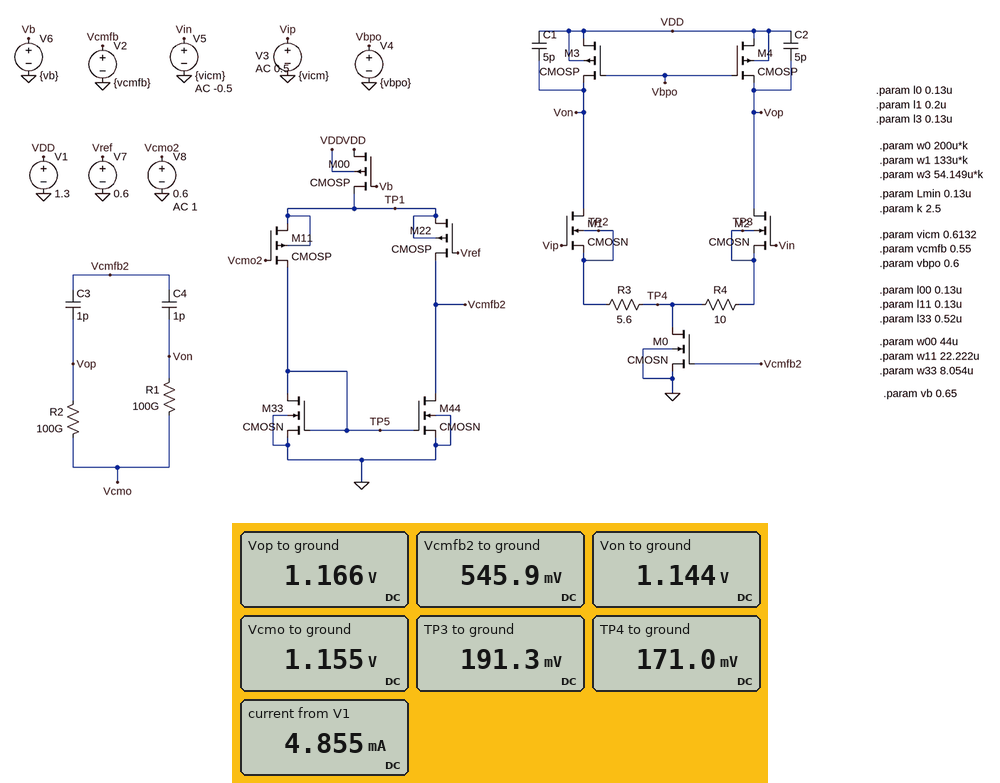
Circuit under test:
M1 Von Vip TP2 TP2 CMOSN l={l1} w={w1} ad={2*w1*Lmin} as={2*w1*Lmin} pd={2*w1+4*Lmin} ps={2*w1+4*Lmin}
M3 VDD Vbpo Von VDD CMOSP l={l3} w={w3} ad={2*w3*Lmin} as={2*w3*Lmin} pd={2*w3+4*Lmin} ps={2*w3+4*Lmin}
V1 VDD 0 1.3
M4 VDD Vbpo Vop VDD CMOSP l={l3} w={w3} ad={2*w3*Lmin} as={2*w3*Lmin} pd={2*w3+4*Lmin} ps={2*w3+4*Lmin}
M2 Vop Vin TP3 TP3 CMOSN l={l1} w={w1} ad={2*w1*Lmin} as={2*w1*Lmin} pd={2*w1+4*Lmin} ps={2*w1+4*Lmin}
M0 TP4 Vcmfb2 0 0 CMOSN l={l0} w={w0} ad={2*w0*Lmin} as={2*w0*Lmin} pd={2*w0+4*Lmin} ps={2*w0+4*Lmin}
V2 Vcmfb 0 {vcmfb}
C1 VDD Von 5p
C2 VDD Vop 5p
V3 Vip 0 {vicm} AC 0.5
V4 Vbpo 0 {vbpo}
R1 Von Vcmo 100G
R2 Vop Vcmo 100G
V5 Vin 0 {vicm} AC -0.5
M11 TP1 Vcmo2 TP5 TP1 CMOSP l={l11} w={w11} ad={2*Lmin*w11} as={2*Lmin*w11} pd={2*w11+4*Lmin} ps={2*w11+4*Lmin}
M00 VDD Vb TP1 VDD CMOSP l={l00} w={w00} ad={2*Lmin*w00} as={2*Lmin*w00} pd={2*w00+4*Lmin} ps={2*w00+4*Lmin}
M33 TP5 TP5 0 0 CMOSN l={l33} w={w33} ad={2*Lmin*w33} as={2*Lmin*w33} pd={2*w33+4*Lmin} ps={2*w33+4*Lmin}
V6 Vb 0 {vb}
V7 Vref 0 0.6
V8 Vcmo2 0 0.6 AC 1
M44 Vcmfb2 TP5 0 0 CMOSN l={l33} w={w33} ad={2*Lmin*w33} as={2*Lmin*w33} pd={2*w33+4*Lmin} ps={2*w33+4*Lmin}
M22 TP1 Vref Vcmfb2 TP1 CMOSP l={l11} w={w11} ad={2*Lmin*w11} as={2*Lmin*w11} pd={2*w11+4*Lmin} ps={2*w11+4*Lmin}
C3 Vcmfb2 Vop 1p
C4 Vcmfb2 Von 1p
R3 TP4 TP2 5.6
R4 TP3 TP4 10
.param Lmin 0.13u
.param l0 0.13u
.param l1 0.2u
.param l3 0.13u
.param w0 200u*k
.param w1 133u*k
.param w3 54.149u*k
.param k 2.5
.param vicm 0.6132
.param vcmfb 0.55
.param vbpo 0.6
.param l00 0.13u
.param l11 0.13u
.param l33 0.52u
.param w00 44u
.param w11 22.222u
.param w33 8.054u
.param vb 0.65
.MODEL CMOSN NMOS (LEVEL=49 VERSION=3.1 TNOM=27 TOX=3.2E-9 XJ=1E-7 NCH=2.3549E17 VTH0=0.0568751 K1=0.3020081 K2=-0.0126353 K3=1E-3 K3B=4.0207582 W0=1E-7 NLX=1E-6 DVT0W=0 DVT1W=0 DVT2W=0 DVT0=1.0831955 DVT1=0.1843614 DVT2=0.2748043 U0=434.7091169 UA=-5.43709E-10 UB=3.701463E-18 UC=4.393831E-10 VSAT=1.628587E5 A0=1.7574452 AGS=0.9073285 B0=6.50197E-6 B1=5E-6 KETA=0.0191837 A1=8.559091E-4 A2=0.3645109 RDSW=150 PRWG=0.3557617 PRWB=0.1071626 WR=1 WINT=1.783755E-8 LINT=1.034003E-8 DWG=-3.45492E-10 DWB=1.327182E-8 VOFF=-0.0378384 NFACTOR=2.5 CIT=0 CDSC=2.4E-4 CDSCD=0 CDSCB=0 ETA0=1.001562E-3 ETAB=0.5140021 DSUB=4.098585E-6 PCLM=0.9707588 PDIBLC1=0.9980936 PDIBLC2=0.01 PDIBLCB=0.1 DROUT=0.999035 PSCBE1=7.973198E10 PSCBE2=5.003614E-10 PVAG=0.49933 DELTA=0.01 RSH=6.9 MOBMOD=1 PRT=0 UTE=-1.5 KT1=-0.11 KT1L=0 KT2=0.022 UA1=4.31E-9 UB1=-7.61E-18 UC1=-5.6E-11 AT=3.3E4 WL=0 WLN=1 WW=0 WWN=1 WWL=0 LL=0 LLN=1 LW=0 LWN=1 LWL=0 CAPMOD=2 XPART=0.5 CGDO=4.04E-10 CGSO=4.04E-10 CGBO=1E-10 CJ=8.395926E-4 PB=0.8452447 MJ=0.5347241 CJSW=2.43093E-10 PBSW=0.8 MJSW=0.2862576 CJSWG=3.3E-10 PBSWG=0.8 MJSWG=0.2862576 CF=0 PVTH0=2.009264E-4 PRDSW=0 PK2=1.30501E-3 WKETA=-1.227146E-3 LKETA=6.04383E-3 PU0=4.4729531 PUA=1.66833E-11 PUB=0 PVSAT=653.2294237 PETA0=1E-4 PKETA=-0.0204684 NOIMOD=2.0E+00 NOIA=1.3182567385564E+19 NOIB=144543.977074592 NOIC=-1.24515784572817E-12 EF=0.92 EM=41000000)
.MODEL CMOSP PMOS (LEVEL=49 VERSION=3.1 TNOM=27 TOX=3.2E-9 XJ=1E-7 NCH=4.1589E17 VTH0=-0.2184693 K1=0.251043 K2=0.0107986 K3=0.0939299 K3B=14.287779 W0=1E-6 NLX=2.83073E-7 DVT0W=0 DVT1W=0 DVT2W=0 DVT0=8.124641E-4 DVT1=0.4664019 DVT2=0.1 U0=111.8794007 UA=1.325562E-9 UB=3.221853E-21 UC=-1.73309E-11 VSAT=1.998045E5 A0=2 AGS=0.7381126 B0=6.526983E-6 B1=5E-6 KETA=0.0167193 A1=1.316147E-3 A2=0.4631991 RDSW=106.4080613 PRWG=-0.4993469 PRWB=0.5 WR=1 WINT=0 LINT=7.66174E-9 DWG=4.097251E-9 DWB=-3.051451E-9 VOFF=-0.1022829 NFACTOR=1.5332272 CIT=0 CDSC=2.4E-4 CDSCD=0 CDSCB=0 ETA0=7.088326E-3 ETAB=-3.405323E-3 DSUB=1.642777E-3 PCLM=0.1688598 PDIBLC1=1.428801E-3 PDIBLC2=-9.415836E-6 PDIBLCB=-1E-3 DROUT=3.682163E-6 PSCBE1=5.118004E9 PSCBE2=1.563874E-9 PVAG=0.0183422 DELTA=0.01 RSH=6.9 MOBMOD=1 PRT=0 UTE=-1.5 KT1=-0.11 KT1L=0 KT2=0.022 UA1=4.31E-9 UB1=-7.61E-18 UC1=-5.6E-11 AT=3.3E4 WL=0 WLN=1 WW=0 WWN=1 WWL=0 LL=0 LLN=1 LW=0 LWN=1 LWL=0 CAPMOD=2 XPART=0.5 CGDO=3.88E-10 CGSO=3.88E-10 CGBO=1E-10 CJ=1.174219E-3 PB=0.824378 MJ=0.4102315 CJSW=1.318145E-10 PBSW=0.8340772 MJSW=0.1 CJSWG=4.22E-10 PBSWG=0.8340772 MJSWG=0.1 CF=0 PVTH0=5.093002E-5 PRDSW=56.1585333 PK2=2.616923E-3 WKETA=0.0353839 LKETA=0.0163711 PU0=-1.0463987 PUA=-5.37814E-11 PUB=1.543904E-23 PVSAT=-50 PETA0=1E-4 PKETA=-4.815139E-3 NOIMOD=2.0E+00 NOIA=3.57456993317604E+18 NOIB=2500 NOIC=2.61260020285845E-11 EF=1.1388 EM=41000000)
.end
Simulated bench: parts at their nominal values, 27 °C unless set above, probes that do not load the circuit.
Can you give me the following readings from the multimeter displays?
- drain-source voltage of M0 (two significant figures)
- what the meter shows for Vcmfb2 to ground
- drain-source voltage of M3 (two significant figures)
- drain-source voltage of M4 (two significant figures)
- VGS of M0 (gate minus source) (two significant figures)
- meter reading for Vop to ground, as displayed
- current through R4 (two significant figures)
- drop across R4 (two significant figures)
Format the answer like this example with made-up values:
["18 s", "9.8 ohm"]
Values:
["170 mV", "545.9 mV", "160 mV", "130 mV", "550 mV", "1.166 V", "2.0 mA", "20 mV"]
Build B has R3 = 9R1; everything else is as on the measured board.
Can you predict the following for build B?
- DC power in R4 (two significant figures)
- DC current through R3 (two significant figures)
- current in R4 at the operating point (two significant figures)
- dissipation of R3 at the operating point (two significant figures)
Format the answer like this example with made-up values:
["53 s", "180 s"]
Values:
["45 µW", "2.2 mA", "2.1 mA", "43 µW"]
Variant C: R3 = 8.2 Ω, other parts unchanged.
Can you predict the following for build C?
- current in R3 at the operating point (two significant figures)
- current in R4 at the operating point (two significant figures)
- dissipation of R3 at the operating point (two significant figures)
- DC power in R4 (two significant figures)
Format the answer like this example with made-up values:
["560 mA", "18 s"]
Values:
["2.2 mA", "2.1 mA", "39 µW", "44 µW"]
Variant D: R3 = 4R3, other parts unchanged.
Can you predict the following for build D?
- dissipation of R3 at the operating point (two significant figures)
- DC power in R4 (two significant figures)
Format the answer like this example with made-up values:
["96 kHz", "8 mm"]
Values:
["23 µW", "40 µW"]
